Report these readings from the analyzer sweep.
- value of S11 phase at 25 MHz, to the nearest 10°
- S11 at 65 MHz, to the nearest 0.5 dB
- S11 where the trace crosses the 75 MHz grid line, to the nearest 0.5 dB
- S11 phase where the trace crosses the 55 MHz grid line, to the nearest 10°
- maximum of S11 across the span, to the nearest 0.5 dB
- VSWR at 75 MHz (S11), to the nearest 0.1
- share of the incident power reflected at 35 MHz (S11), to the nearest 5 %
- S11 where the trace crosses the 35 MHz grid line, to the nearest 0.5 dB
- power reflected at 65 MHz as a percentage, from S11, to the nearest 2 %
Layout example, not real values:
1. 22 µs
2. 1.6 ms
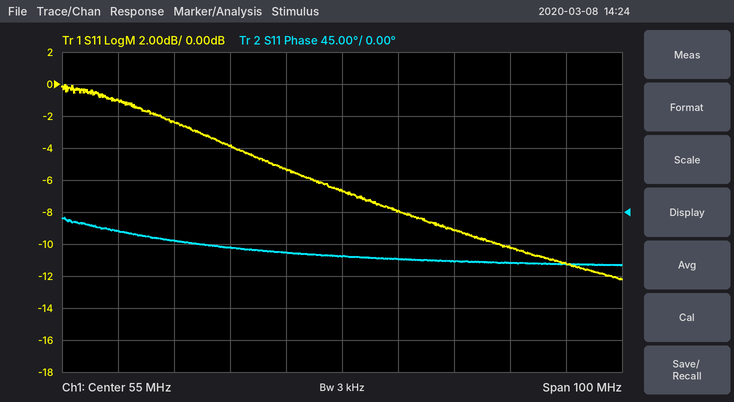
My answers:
1. -40°
2. -8.0 dB
3. -9.0 dB
4. -60°
5. 0.0 dB
6. 2.1
7. 40 %
8. -4.0 dB
9. 16 %
